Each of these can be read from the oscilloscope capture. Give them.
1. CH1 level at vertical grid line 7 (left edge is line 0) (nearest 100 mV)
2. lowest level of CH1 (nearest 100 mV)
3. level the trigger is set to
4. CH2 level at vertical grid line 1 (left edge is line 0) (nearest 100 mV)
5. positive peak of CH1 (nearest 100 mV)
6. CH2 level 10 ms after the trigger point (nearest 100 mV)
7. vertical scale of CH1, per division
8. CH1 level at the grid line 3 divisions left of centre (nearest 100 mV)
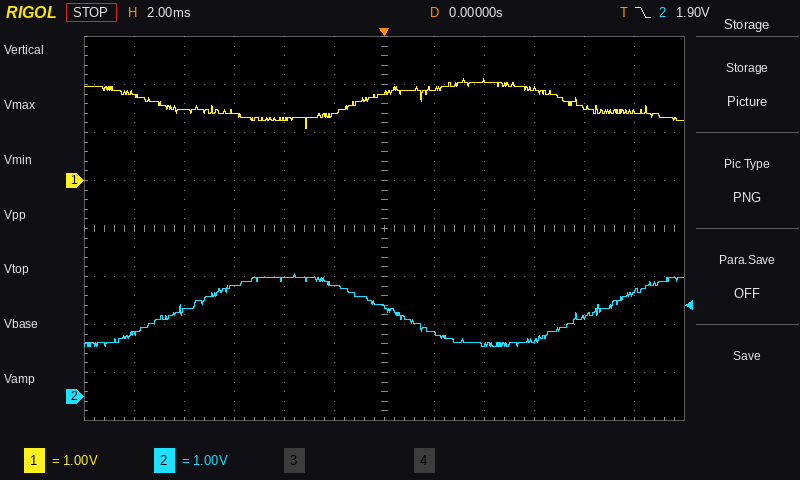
1.9 V
1.1 V
1.90 V
1.3 V
2.1 V
2.2 V
1 V
1.4 V
